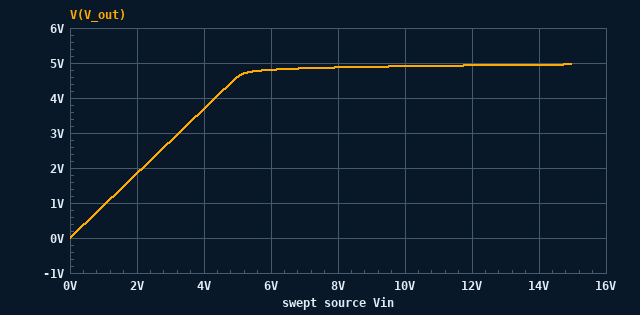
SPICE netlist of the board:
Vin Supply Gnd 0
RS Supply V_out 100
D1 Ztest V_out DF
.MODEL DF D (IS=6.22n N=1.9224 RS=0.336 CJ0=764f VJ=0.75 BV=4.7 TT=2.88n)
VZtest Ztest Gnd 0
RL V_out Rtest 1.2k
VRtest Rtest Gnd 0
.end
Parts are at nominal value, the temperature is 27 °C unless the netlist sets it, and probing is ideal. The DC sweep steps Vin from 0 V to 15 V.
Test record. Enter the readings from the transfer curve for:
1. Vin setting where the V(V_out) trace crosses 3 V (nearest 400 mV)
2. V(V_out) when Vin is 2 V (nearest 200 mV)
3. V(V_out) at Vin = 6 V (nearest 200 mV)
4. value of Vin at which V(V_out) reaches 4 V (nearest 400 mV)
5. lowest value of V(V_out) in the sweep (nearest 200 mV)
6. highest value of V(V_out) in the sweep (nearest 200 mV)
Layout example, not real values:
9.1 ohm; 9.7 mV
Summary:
3.2 V; 1.8 V; 4.8 V; 4.4 V; 0 V; 5.0 V
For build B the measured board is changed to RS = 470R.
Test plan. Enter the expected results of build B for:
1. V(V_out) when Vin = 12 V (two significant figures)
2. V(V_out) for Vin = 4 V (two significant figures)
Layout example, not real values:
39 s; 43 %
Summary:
4.8 V; 2.9 V
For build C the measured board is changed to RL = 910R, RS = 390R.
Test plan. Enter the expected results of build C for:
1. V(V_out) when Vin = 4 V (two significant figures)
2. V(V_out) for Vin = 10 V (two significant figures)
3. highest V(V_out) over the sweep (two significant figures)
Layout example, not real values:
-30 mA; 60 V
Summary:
2.8 V; 4.8 V; 4.9 V
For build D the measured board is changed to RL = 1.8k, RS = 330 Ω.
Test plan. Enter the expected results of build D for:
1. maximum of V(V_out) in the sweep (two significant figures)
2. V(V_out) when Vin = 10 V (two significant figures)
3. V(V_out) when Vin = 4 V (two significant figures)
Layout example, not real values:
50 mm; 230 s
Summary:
4.9 V; 4.8 V; 3.4 V
